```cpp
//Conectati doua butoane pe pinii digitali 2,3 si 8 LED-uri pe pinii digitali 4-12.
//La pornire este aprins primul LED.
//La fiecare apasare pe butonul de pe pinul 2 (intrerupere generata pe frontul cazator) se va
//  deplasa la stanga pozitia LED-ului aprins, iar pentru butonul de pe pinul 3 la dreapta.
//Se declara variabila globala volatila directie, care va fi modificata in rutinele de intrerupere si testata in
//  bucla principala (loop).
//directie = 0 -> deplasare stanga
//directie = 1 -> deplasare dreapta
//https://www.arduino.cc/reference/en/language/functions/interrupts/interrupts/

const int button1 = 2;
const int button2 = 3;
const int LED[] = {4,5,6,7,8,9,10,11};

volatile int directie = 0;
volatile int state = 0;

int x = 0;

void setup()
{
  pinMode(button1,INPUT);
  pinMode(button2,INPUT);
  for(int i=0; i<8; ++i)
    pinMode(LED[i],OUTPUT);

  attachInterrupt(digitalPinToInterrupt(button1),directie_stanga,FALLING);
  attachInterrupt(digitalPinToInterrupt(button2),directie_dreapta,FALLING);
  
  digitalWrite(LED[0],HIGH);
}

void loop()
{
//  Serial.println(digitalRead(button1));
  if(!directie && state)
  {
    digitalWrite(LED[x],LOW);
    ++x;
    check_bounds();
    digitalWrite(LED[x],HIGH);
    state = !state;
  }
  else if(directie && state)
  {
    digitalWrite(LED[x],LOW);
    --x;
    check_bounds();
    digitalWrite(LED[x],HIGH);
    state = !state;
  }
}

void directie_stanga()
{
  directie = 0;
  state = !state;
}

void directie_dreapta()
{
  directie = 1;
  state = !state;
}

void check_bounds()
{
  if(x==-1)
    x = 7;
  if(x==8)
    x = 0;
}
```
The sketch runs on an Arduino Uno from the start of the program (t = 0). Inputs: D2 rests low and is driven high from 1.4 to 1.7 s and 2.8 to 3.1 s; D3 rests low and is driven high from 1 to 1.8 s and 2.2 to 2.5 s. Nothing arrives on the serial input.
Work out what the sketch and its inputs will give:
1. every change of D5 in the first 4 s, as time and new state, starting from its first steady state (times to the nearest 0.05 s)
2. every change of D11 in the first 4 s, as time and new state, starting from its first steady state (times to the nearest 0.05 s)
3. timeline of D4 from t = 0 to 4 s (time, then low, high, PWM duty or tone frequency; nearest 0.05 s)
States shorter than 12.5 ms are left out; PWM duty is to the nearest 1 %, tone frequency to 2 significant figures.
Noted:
0 s low; 1.7 s high; 1.8 s low
0 s low; 2.5 s high; 3.1 s low
0 s high; 1.7 s low; 1.8 s high; 2.5 s low; 3.1 s high
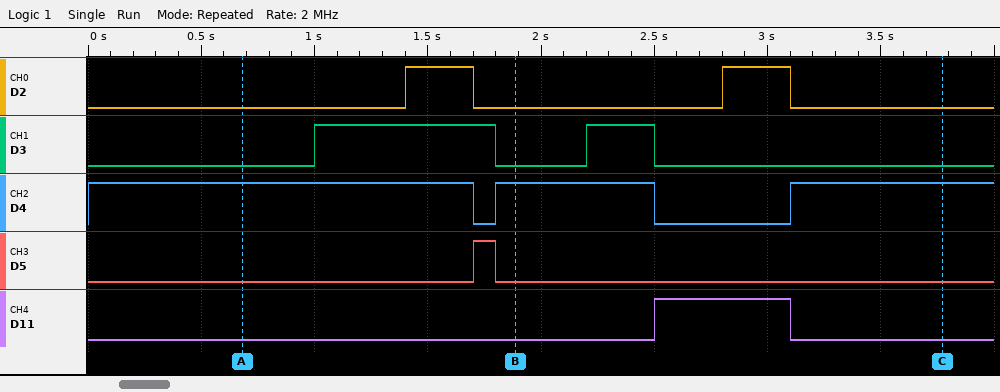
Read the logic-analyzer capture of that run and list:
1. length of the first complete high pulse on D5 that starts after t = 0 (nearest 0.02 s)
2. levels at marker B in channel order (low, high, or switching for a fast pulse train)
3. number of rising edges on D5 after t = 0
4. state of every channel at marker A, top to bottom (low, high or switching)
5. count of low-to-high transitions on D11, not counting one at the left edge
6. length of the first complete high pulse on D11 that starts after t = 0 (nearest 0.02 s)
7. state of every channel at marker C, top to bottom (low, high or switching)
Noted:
0.10 s
D2 low, D3 low, D4 high, D5 low, D11 low
1
D2 low, D3 low, D4 high, D5 low, D11 low
1
0.60 s
D2 low, D3 low, D4 high, D5 low, D11 low
